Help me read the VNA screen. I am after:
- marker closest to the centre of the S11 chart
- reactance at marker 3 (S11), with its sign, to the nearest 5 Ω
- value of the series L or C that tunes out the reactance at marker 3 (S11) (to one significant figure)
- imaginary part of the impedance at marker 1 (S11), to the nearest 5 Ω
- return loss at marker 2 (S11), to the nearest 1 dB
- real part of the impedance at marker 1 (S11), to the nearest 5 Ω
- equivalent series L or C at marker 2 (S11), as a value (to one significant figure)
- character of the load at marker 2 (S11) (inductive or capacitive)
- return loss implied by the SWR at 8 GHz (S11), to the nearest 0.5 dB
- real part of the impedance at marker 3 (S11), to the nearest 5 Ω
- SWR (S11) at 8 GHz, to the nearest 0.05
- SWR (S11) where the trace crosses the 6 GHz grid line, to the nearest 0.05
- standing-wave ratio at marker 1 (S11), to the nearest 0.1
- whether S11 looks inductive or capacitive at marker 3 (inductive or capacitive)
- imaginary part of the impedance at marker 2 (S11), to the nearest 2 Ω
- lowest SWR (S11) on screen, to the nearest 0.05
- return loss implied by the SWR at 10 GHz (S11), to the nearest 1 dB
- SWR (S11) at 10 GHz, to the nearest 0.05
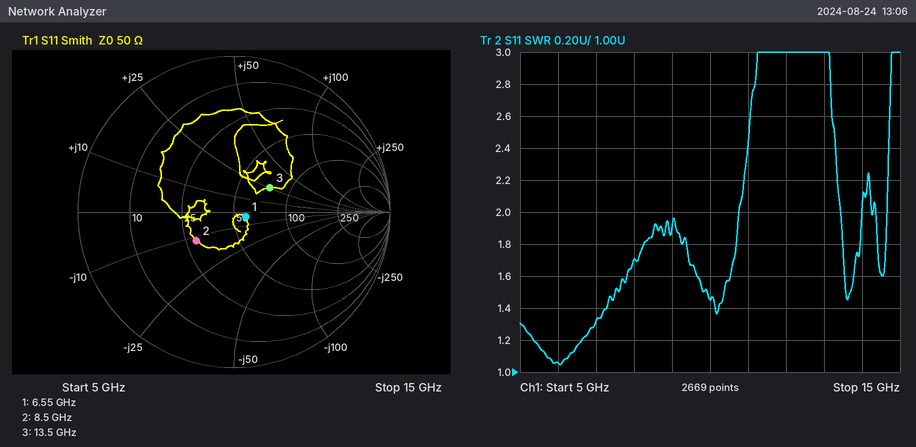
marker 1
+25 Ω
500 fF
-5 Ω
10 dB
60 Ω
2 pF
capacitive
11.5 dB
75 Ω
1.70
1.05
1.2
inductive
-12 Ω
1.05
15 dB
1.45
